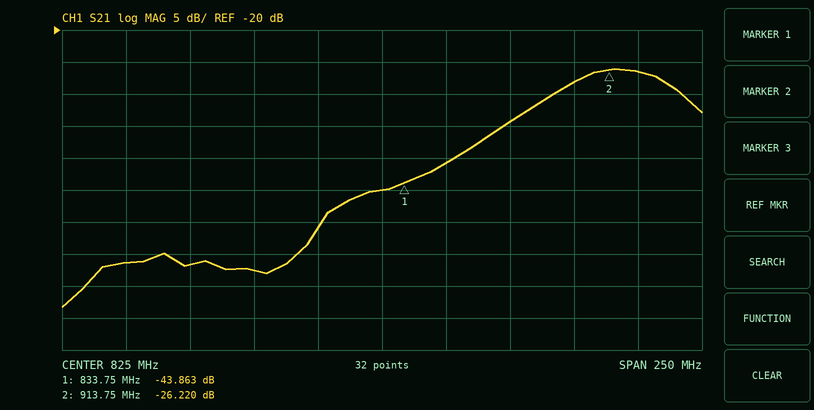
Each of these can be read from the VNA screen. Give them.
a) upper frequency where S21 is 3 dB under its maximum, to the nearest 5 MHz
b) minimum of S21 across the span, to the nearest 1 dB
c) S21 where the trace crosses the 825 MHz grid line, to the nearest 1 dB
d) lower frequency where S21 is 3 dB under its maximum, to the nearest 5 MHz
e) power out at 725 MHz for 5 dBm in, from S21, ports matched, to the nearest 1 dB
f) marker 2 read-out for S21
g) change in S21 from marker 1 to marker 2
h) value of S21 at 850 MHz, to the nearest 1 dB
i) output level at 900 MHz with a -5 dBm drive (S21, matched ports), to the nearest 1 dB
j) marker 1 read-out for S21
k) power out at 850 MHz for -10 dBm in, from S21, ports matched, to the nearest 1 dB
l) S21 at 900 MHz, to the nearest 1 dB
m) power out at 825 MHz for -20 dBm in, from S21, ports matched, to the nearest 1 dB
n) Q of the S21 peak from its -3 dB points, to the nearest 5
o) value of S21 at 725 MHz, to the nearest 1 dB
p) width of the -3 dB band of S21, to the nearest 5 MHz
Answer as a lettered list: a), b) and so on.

a) 940 MHz
b) -63 dB
c) -45 dB
d) 895 MHz
e) -51 dBm
f) -26.220 dB
g) 17.643 dB
h) -41 dB
i) -33 dBm
j) -43.863 dB
k) -51 dBm
l) -28 dB
m) -65 dBm
n) 20
o) -56 dB
p) 45 MHz
